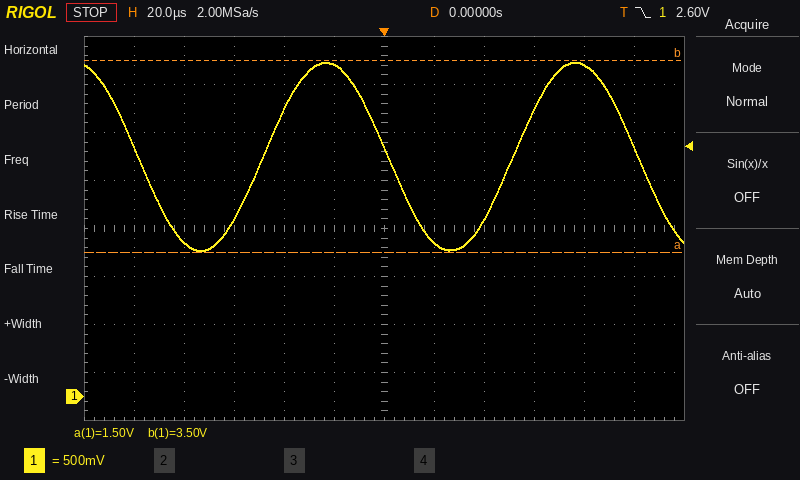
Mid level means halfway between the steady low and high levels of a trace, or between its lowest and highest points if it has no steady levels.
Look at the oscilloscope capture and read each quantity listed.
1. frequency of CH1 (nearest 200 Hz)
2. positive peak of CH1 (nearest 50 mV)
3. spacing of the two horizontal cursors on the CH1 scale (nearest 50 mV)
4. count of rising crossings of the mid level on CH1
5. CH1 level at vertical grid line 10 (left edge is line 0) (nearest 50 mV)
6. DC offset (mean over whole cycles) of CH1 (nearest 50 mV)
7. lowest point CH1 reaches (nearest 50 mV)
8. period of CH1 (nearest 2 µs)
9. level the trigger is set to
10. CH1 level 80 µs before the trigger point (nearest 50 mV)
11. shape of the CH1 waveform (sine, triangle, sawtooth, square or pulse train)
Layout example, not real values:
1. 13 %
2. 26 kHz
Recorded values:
1. 10.0 kHz
2. 3.50 V
3. 2.00 V
4. 2
5. 3.45 V
6. 2.50 V
7. 1.50 V
8. 100 µs
9. 2.60 V
10. 1.60 V
11. sine
